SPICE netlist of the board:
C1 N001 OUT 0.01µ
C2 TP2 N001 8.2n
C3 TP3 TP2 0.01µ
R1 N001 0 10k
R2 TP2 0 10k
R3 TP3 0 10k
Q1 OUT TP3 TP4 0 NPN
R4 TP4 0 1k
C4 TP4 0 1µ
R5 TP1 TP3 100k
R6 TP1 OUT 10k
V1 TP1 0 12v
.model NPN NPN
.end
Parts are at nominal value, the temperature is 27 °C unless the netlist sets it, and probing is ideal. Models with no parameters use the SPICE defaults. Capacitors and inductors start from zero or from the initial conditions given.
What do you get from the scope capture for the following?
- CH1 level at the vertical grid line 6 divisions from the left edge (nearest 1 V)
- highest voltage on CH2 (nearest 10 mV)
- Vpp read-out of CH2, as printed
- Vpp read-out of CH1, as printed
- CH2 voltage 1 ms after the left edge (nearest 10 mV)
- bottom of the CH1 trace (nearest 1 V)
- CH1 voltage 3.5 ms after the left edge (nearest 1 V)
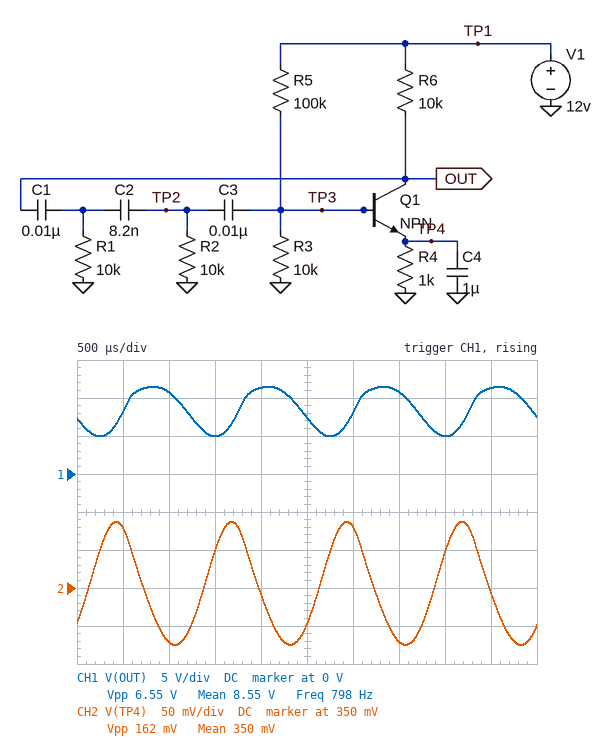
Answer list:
8 V
440 mV
162 mV
6.55 V
280 mV
5 V
11 V
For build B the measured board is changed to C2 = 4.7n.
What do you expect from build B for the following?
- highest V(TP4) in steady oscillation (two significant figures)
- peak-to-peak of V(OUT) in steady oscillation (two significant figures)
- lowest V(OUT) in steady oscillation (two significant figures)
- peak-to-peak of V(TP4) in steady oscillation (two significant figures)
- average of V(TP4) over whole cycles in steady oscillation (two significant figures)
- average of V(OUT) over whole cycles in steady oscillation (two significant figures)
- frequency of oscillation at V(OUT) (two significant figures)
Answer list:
410 mV
5.9 V
5.4 V
130 mV
340 mV
8.6 V
940 Hz
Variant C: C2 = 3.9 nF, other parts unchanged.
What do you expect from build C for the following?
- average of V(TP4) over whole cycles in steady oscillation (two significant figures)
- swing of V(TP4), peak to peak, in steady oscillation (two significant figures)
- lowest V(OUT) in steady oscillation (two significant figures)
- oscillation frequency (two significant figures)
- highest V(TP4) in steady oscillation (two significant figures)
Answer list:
340 mV
120 mV
5.6 V
1.0 kHz
400 mV
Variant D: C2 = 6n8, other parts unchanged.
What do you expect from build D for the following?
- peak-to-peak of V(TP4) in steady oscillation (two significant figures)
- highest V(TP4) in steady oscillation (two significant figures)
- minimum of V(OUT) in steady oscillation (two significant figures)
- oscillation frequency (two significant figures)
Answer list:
150 mV
430 mV
5.1 V
840 Hz
